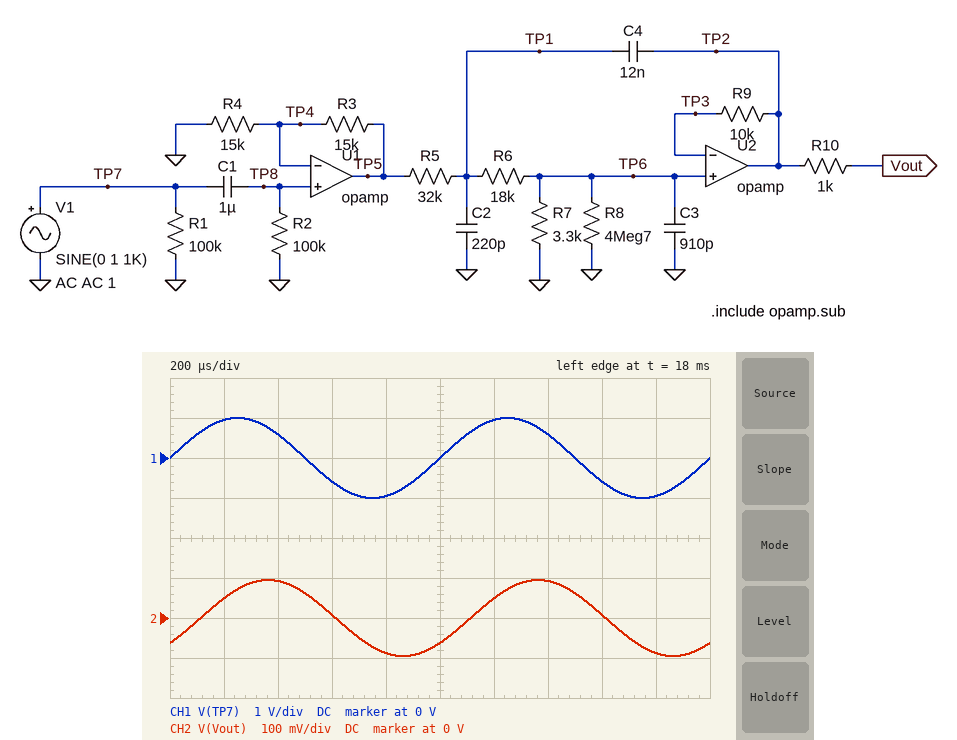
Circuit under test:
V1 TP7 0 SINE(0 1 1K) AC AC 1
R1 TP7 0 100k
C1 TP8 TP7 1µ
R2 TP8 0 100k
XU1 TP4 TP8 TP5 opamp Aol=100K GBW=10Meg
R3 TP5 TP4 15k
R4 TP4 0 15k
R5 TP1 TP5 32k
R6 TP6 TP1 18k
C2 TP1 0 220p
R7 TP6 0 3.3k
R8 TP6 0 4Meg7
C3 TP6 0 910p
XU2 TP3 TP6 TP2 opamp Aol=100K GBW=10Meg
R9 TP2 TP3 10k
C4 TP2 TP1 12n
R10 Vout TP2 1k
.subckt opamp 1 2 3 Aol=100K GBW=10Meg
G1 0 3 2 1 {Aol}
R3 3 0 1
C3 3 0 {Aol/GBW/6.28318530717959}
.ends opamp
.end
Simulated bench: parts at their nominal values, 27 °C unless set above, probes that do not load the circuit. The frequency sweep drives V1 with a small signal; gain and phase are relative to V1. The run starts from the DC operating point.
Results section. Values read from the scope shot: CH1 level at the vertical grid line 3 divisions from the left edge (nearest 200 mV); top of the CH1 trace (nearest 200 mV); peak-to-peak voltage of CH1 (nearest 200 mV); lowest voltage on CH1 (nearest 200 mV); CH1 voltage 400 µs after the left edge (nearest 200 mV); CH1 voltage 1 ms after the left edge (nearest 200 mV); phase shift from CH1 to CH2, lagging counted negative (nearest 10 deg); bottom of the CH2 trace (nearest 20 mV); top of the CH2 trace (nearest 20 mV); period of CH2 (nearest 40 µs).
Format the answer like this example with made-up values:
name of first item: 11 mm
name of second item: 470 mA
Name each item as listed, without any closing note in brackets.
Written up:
CH1 level at the vertical grid line 3 divisions from the left edge: -600 mV
top of the CH1 trace: 1.0 V
peak-to-peak voltage of CH1: 2.0 V
lowest voltage on CH1: -1.0 V
CH1 voltage 400 µs after the left edge: 600 mV
CH1 voltage 1 ms after the left edge: 0 V
phase shift from CH1 to CH2, lagging counted negative: -40 deg
bottom of the CH2 trace: -100 mV
top of the CH2 trace: 100 mV
period of CH2: 1.00 ms
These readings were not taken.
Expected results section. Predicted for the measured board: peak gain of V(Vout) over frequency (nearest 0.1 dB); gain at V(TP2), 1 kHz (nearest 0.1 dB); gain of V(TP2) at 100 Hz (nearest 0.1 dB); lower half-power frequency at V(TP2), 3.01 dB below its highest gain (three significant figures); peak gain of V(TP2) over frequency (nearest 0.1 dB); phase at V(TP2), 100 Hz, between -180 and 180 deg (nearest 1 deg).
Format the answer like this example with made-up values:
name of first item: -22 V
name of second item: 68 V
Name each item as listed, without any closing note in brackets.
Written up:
peak gain of V(Vout) over frequency: -18.2 dB
gain at V(TP2), 1 kHz: -20.4 dB
gain of V(TP2) at 100 Hz: -18.2 dB
lower half-power frequency at V(TP2), 3.01 dB below its highest gain: 1.59 Hz
peak gain of V(TP2) over frequency: -18.2 dB
phase at V(TP2), 100 Hz, between -180 and 180 deg: -4 deg
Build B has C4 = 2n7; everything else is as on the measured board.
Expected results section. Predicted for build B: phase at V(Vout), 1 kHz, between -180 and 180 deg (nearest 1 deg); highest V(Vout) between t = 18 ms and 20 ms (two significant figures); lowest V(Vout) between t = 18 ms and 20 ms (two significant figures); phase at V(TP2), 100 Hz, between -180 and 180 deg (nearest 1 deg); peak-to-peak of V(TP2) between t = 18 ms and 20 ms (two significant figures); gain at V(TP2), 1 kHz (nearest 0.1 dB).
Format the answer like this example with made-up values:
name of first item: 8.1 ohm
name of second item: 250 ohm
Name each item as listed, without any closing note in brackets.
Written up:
phase at V(Vout), 1 kHz, between -180 and 180 deg: -12 deg
highest V(Vout) between t = 18 ms and 20 ms: 120 mV
lowest V(Vout) between t = 18 ms and 20 ms: -120 mV
phase at V(TP2), 100 Hz, between -180 and 180 deg: 0 deg
peak-to-peak of V(TP2) between t = 18 ms and 20 ms: 240 mV
gain at V(TP2), 1 kHz: -18.3 dB
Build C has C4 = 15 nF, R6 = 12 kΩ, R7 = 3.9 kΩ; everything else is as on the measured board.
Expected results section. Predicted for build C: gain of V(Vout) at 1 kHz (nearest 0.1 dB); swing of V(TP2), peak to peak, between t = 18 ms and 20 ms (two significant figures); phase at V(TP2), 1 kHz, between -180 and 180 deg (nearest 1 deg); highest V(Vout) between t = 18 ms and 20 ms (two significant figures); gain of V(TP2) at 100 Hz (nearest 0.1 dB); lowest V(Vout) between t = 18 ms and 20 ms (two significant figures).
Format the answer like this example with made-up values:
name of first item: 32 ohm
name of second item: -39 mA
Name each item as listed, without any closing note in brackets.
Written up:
gain of V(Vout) at 1 kHz: -17.8 dB
swing of V(TP2), peak to peak, between t = 18 ms and 20 ms: 260 mV
phase at V(TP2), 1 kHz, between -180 and 180 deg: -39 deg
highest V(Vout) between t = 18 ms and 20 ms: 130 mV
gain of V(TP2) at 100 Hz: -15.8 dB
lowest V(Vout) between t = 18 ms and 20 ms: -130 mV
